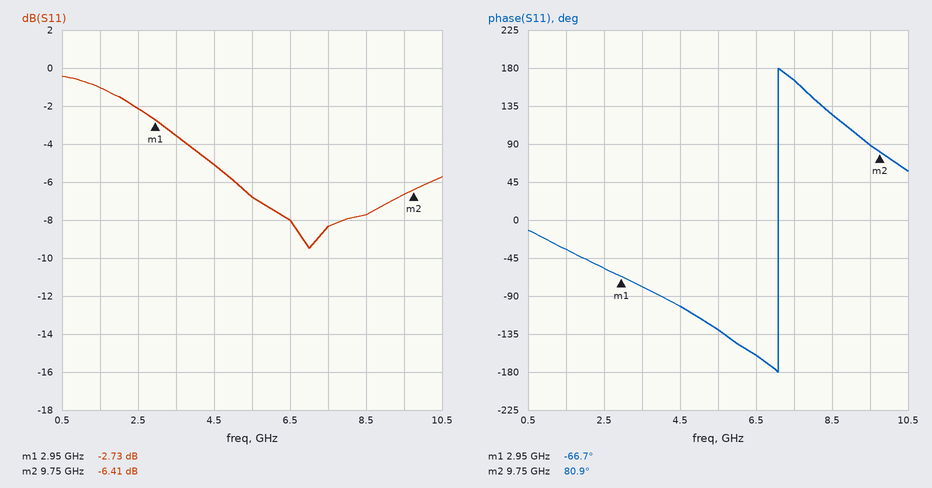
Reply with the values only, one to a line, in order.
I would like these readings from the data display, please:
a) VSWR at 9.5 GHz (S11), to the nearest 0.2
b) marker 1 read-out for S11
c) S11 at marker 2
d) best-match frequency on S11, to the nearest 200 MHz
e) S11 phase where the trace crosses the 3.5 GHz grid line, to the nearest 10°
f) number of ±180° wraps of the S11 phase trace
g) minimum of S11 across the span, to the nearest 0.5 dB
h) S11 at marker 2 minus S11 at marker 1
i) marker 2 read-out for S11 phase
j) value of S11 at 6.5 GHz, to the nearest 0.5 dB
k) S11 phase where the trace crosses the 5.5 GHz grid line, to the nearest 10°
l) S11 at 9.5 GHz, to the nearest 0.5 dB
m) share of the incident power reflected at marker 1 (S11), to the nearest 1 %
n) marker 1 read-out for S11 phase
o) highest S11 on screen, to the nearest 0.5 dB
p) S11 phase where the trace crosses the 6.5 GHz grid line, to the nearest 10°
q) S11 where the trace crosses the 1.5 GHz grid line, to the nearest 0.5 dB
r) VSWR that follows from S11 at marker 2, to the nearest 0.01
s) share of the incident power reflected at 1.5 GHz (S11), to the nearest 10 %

2.8
-2.73 dB
-6.41 dB
7.0 GHz
-80°
1
-9.5 dB
-3.68 dB
80.9°
-8.0 dB
-130°
-6.5 dB
53 %
-66.7°
-0.5 dB
-160°
-1.0 dB
2.83
80 %
